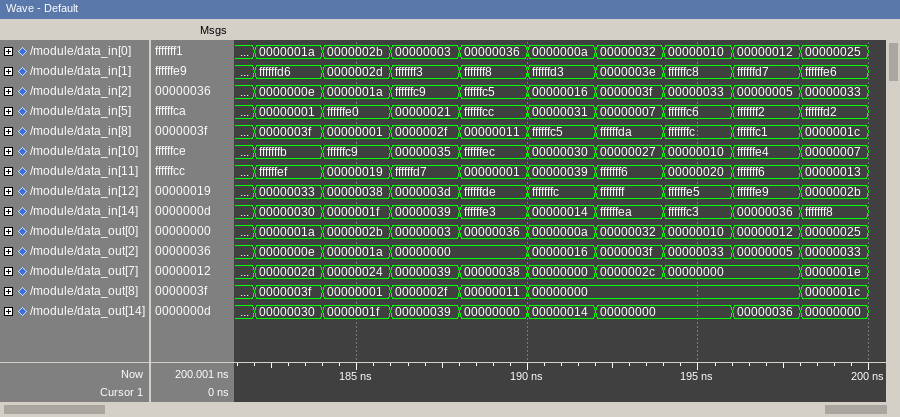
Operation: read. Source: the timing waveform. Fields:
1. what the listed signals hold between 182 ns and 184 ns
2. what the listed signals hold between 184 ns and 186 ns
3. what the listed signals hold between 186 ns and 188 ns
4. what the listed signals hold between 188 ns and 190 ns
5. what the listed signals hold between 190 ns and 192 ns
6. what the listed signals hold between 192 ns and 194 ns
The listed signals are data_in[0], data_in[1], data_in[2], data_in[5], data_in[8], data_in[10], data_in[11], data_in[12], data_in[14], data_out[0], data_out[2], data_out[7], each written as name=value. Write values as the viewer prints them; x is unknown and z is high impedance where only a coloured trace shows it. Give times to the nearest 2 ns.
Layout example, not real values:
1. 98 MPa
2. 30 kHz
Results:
1. data_in[0]=0000001a, data_in[1]=ffffffd6, data_in[2]=0000000e, data_in[5]=00000001, data_in[8]=0000003f, data_in[10]=fffffffb, data_in[11]=ffffffef, data_in[12]=00000033, data_in[14]=00000030, data_out[0]=0000001a, data_out[2]=0000000e, data_out[7]=0000002d
2. data_in[0]=0000002b, data_in[1]=0000002d, data_in[2]=0000001a, data_in[5]=ffffffe0, data_in[8]=00000001, data_in[10]=ffffffc9, data_in[11]=00000019, data_in[12]=00000038, data_in[14]=0000001f, data_out[0]=0000002b, data_out[2]=0000001a, data_out[7]=00000024
3. data_in[0]=00000003, data_in[1]=fffffff3, data_in[2]=ffffffc9, data_in[5]=00000021, data_in[8]=0000002f, data_in[10]=00000035, data_in[11]=ffffffd7, data_in[12]=0000003d, data_in[14]=00000039, data_out[0]=00000003, data_out[2]=00000000, data_out[7]=00000039
4. data_in[0]=00000036, data_in[1]=fffffff8, data_in[2]=ffffffc5, data_in[5]=ffffffcc, data_in[8]=00000011, data_in[10]=ffffffec, data_in[11]=00000001, data_in[12]=ffffffde, data_in[14]=ffffffe3, data_out[0]=00000036, data_out[2]=00000000, data_out[7]=00000038
5. data_in[0]=0000000a, data_in[1]=ffffffd3, data_in[2]=00000016, data_in[5]=00000031, data_in[8]=ffffffc5, data_in[10]=00000030, data_in[11]=00000039, data_in[12]=fffffffc, data_in[14]=00000014, data_out[0]=0000000a, data_out[2]=00000016, data_out[7]=00000000
6. data_in[0]=00000032, data_in[1]=0000003e, data_in[2]=0000003f, data_in[5]=00000007, data_in[8]=ffffffda, data_in[10]=00000027, data_in[11]=fffffff6, data_in[12]=ffffffff, data_in[14]=ffffffea, data_out[0]=00000032, data_out[2]=0000003f, data_out[7]=0000002c
